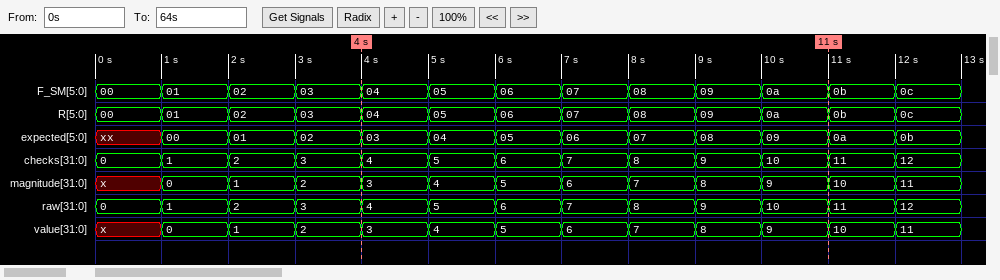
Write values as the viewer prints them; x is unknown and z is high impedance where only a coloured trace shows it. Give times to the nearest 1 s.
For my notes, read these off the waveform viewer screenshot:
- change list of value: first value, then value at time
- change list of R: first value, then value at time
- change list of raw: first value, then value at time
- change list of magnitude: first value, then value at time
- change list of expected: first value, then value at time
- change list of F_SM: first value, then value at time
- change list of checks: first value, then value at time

x, 0 at 1 s, 1 at 2 s, 2 at 3 s, 3 at 4 s, 4 at 5 s, 5 at 6 s, 6 at 7 s, 7 at 8 s, 8 at 9 s, 9 at 10 s, 10 at 11 s, 11 at 12 s
00, 01 at 1 s, 02 at 2 s, 03 at 3 s, 04 at 4 s, 05 at 5 s, 06 at 6 s, 07 at 7 s, 08 at 8 s, 09 at 9 s, 0a at 10 s, 0b at 11 s, 0c at 12 s
0, 1 at 1 s, 2 at 2 s, 3 at 3 s, 4 at 4 s, 5 at 5 s, 6 at 6 s, 7 at 7 s, 8 at 8 s, 9 at 9 s, 10 at 10 s, 11 at 11 s, 12 at 12 s
x, 0 at 1 s, 1 at 2 s, 2 at 3 s, 3 at 4 s, 4 at 5 s, 5 at 6 s, 6 at 7 s, 7 at 8 s, 8 at 9 s, 9 at 10 s, 10 at 11 s, 11 at 12 s
xx, 00 at 1 s, 01 at 2 s, 02 at 3 s, 03 at 4 s, 04 at 5 s, 05 at 6 s, 06 at 7 s, 07 at 8 s, 08 at 9 s, 09 at 10 s, 0a at 11 s, 0b at 12 s
00, 01 at 1 s, 02 at 2 s, 03 at 3 s, 04 at 4 s, 05 at 5 s, 06 at 6 s, 07 at 7 s, 08 at 8 s, 09 at 9 s, 0a at 10 s, 0b at 11 s, 0c at 12 s
0, 1 at 1 s, 2 at 2 s, 3 at 3 s, 4 at 4 s, 5 at 5 s, 6 at 6 s, 7 at 7 s, 8 at 8 s, 9 at 9 s, 10 at 10 s, 11 at 11 s, 12 at 12 s
